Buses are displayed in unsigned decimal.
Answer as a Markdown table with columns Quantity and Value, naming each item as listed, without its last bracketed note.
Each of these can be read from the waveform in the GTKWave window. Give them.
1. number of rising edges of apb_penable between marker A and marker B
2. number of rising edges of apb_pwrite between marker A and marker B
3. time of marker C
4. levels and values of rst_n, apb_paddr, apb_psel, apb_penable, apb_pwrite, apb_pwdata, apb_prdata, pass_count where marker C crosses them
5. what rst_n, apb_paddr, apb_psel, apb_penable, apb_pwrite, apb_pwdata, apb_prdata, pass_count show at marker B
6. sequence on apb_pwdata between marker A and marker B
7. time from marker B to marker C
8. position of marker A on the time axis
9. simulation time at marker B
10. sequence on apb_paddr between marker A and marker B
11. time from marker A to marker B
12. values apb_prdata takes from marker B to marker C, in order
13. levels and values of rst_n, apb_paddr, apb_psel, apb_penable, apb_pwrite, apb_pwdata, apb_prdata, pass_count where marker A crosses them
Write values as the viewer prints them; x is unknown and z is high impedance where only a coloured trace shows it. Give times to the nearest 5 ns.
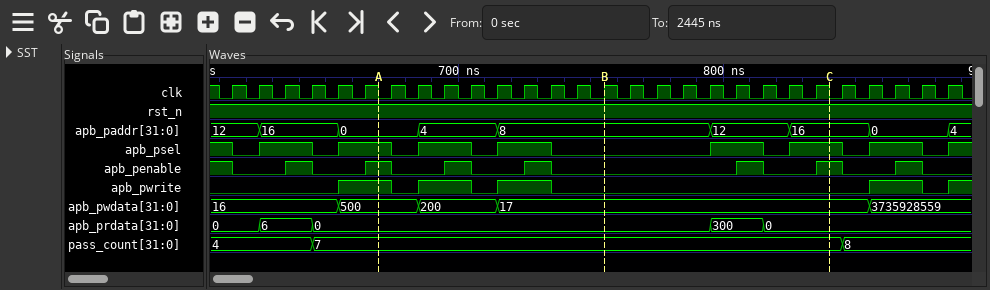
| Quantity | Value |
|---|---|
| number of rising edges of apb_penable between marker A and marker B | 2 |
| number of rising edges of apb_pwrite between marker A and marker B | 2 |
| time of marker C | 840 ns |
| levels and values of rst_n, apb_paddr, apb_psel, apb_penable, apb_pwrite, apb_pwdata, apb_prdata, pass_count where marker C crosses them | rst_n=1, apb_paddr=16, apb_psel=1, apb_penable=1, apb_pwrite=0, apb_pwdata=17, apb_prdata=0, pass_count=7 |
| what rst_n, apb_paddr, apb_psel, apb_penable, apb_pwrite, apb_pwdata, apb_prdata, pass_count show at marker B | rst_n=1, apb_paddr=8, apb_psel=0, apb_penable=0, apb_pwrite=0, apb_pwdata=17, apb_prdata=0, pass_count=7 |
| sequence on apb_pwdata between marker A and marker B | 500, 200, 17 |
| time from marker B to marker C | 85 ns |
| position of marker A on the time axis | 670 ns |
| simulation time at marker B | 755 ns |
| sequence on apb_paddr between marker A and marker B | 0, 4, 8 |
| time from marker A to marker B | 85 ns |
| values apb_prdata takes from marker B to marker C, in order | 0, 300, 0 |
| levels and values of rst_n, apb_paddr, apb_psel, apb_penable, apb_pwrite, apb_pwdata, apb_prdata, pass_count where marker A crosses them | rst_n=1, apb_paddr=0, apb_psel=1, apb_penable=1, apb_pwrite=1, apb_pwdata=500, apb_prdata=0, pass_count=7 |
